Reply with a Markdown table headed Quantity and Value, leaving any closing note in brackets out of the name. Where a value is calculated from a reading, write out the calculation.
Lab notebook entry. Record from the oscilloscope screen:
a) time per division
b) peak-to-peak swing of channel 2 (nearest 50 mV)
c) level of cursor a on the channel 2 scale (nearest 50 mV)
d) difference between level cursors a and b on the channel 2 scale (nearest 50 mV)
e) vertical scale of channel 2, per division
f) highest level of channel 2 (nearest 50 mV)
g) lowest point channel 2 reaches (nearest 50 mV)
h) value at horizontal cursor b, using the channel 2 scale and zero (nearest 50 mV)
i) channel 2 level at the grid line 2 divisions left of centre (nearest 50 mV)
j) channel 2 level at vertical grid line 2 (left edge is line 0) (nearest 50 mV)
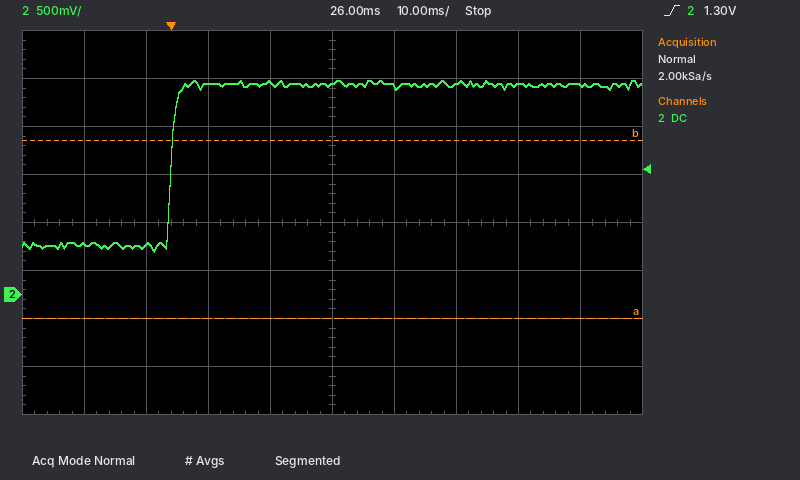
| Quantity | Value |
|---|---|
| time per division | 10 ms |
| peak-to-peak swing of channel 2 | 2.25 V − (450 mV) = 1.80 V |
| level of cursor a on the channel 2 scale | -250 mV |
| difference between level cursors a and b on the channel 2 scale | 1.85 V |
| vertical scale of channel 2, per division | 500 mV |
| highest level of channel 2 | 2.25 V |
| lowest point channel 2 reaches | 450 mV |
| value at horizontal cursor b, using the channel 2 scale and zero | 1.60 V |
| channel 2 level at the grid line 2 divisions left of centre | 2.20 V |
| channel 2 level at vertical grid line 2 (left edge is line 0) | 500 mV |
